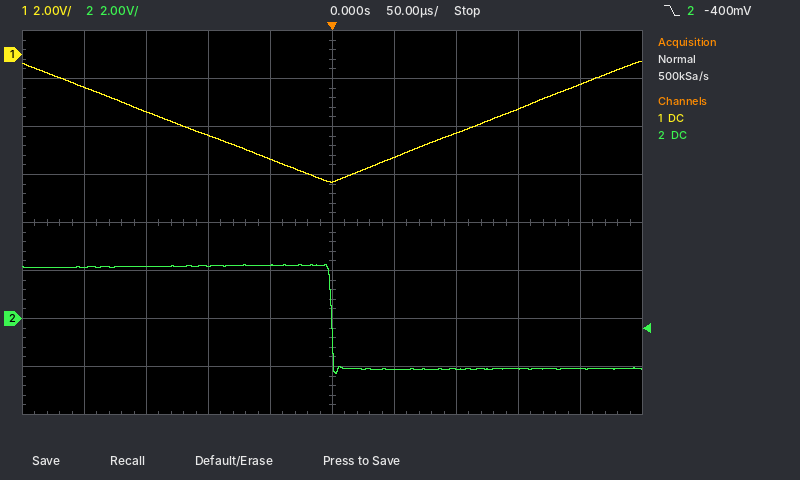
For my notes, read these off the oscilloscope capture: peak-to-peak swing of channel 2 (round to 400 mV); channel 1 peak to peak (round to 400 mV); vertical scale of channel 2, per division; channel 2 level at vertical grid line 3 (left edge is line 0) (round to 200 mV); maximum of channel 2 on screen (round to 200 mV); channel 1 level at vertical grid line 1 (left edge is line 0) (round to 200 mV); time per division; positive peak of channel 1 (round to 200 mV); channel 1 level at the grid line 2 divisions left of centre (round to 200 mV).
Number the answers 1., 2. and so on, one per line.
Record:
1. 4.4 V
2. 5.2 V
3. 2 V
4. 2.2 V
5. 2.2 V
6. -1.4 V
7. 50 µs
8. -200 mV
9. -3.4 V
